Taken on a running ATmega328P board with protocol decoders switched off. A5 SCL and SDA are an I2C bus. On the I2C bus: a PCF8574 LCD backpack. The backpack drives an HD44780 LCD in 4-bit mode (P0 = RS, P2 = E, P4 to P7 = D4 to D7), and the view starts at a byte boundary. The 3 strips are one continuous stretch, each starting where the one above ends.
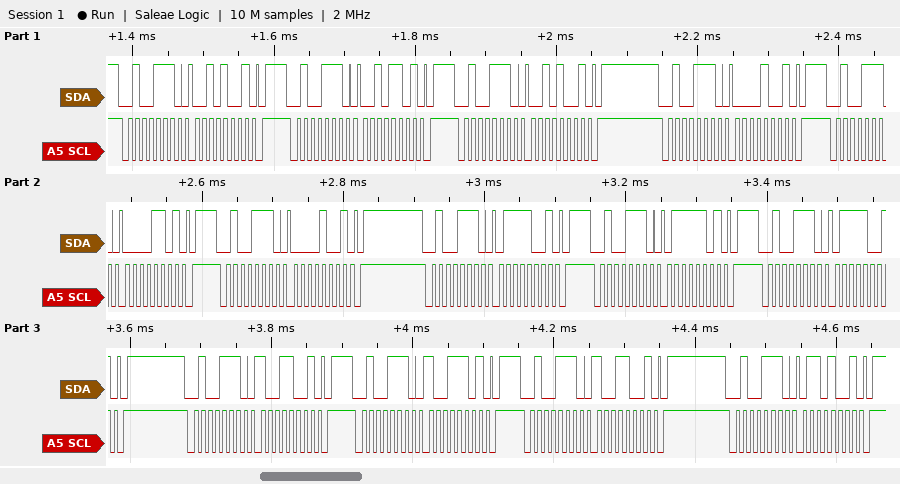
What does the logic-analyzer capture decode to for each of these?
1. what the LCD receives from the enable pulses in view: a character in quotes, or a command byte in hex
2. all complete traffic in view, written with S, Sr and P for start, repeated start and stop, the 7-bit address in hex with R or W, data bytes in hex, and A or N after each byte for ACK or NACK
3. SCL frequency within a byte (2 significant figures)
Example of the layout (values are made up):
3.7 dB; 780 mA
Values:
' ' 'y'; S 27W A 29 A P S 27W A 2D A P S 27W A 29 A P S 27W A 09 A P S 27W A 0D A P S 27W A 09 A P S 27W A 79 A P S 27W A 7D A P S 27W A 79 A P S 27W A 99 A P S 27W A 9D A P S 27W A 99 A P S 27W A 69 A P; 100 kHz
